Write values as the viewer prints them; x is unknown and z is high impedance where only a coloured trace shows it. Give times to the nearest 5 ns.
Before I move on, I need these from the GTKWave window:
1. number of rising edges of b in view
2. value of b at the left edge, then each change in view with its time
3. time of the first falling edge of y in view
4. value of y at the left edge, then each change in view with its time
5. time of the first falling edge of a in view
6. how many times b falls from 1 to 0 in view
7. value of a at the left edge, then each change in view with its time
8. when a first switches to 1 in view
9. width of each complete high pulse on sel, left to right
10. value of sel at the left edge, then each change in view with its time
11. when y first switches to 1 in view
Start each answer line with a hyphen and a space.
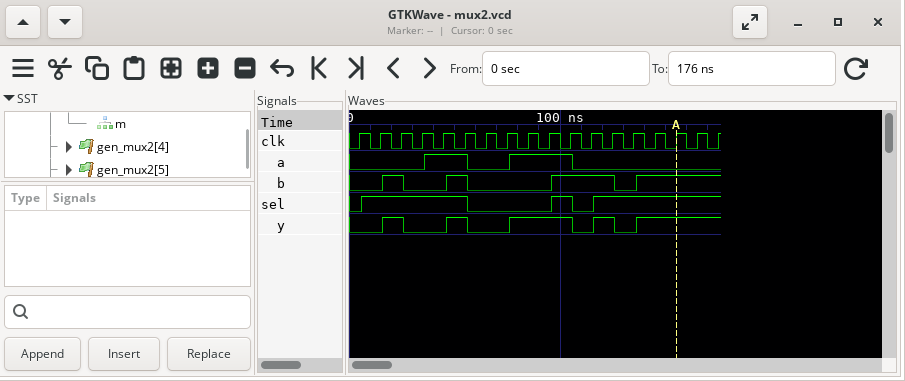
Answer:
- 4
- 0, 1 at 15 ns, 0 at 25 ns, 1 at 45 ns, 0 at 55 ns, 1 at 95 ns, 0 at 125 ns, 1 at 135 ns
- 25 ns
- 0, 1 at 15 ns, 0 at 25 ns, 1 at 45 ns, 0 at 55 ns, 1 at 75 ns, 0 at 105 ns, 1 at 115 ns, 0 at 125 ns, 1 at 135 ns
- 55 ns
- 3
- 0, 1 at 35 ns, 0 at 55 ns, 1 at 75 ns, 0 at 105 ns
- 35 ns
- 50 ns, 10 ns
- 0, 1 at 5 ns, 0 at 55 ns, 1 at 95 ns, 0 at 105 ns, 1 at 115 ns
- 15 ns
